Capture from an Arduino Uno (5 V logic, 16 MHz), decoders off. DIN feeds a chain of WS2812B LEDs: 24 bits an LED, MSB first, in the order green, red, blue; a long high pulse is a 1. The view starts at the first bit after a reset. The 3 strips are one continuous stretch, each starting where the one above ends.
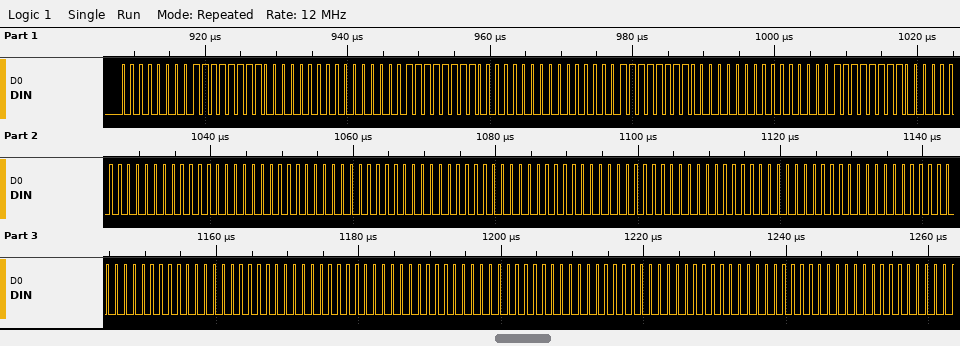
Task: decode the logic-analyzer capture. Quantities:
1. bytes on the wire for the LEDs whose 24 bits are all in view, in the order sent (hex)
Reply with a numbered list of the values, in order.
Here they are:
1. 00 FF 00 00 FF 00 00 FF 00 00 FF 00 00 00 00 00 00 00 00 00 00 00 00 00 00 00 00 00 00 00 00 00 00
